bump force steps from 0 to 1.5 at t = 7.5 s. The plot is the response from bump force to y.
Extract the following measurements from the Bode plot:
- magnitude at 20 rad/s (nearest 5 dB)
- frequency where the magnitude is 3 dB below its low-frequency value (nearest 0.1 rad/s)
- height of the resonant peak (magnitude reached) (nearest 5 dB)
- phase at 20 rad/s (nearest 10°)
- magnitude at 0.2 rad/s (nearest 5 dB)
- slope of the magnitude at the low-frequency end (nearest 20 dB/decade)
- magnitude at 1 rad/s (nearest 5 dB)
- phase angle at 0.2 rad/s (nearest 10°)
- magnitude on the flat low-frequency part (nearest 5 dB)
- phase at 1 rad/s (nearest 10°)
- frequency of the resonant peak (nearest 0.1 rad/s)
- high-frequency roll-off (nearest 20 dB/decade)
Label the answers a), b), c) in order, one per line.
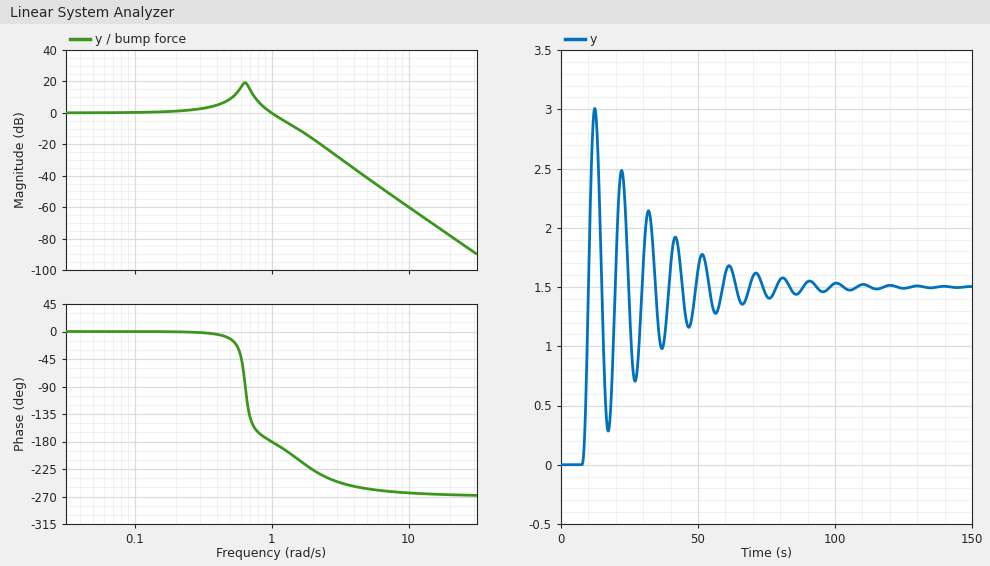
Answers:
a) -80 dB
b) 1.1 rad/s
c) 20 dB
d) -270°
e) 0 dB
f) 0 dB/decade
g) 0 dB
h) 0°
i) 0 dB
j) -180°
k) 0.6 rad/s
l) -60 dB/decade
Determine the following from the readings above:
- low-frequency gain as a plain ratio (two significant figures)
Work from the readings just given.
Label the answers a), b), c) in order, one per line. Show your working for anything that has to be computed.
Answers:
a) 10^(0 / 20) = 1.0
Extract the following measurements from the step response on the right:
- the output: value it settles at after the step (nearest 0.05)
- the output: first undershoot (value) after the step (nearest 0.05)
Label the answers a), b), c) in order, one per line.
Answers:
a) 1.50
b) 0.30
